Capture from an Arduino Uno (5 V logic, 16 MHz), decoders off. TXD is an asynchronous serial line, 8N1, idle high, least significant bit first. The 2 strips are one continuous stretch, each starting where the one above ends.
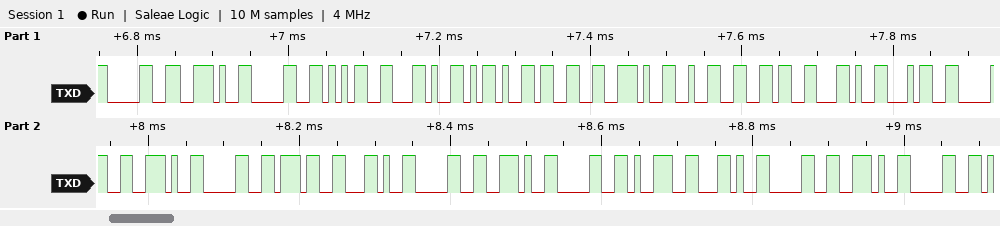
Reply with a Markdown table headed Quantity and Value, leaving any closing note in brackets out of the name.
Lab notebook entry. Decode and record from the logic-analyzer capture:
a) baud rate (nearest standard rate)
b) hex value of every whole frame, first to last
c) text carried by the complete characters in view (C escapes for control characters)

| Quantity | Value |
|---|---|
| baud rate | 115200 baud |
| hex value of every whole frame, first to last | 30 2E 30 35 2C 2D 33 2E 32 36 2C 34 30 2E 30 37 2C 30 2E 30 39 2C 30 2E 30 |
| text carried by the complete characters in view | "0.05,-3.26,40.07,0.09,0.0" |
